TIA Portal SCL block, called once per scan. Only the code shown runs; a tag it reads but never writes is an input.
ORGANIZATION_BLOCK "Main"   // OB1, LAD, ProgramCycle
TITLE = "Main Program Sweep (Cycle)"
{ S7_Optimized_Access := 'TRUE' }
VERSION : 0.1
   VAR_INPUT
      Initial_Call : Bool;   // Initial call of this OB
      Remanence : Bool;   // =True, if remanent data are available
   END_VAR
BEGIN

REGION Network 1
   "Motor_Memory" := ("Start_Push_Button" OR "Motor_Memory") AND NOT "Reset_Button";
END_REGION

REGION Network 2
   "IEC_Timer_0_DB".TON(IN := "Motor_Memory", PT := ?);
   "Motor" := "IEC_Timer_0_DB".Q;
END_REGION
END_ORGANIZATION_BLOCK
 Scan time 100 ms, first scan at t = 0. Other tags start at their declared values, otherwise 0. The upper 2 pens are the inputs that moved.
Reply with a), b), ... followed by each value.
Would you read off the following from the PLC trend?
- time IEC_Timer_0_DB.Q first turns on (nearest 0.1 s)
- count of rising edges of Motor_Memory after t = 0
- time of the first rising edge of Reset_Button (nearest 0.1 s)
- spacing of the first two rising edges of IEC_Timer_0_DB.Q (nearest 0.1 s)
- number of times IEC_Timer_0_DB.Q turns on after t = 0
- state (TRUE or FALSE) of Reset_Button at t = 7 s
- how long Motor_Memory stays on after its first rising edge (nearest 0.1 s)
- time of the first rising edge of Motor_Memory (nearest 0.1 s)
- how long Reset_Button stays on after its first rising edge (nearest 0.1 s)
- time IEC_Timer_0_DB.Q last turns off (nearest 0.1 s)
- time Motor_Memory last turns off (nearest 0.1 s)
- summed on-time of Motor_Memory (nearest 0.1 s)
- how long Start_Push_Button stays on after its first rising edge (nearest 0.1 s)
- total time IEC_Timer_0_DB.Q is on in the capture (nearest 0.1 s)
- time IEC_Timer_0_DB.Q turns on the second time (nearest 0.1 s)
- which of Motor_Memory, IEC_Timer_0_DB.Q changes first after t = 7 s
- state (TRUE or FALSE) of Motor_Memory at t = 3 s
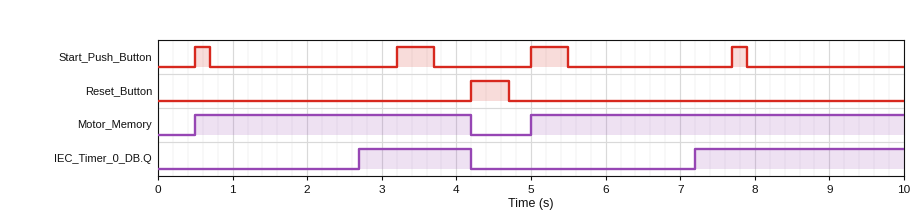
a) 2.7 s
b) 2
c) 4.2 s
d) 4.5 s
e) 2
f) FALSE
g) 3.7 s
h) 0.5 s
i) 0.5 s
j) 4.2 s
k) 4.2 s
l) 8.7 s
m) 0.2 s
n) 4.3 s
o) 7.2 s
p) IEC_Timer_0_DB.Q
q) TRUE
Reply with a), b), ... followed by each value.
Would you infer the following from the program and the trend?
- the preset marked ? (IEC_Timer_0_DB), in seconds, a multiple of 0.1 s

a) 2.2 s
